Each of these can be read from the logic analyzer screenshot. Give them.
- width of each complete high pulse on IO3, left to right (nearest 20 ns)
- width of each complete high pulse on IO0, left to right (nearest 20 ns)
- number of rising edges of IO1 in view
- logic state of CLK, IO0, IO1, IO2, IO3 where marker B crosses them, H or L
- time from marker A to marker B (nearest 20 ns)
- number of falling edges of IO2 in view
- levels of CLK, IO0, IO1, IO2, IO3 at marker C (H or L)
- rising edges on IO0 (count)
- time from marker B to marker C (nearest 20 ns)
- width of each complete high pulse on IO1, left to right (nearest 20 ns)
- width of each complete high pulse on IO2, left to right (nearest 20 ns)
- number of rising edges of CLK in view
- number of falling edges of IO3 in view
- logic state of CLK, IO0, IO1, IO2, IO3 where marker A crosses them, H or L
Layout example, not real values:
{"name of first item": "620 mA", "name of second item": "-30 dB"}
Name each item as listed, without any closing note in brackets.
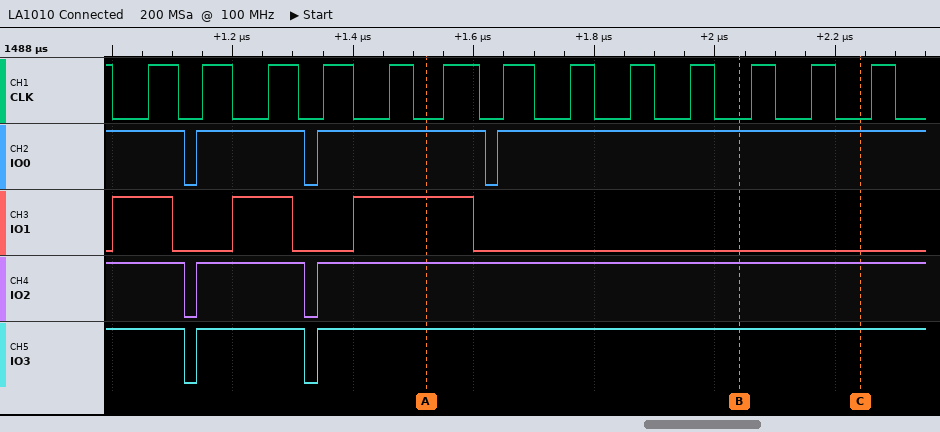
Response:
{"width of each complete high pulse on IO3, left to right": "180 ns", "width of each complete high pulse on IO0, left to right": "180 ns, 280 ns", "number of rising edges of IO1 in view": "3", "logic state of CLK, IO0, IO1, IO2, IO3 where marker B crosses them, H or L": "CLK=L, IO0=H, IO1=L, IO2=H, IO3=H", "time from marker A to marker B": "520 ns", "number of falling edges of IO2 in view": "2", "levels of CLK, IO0, IO1, IO2, IO3 at marker C": "CLK=L, IO0=H, IO1=L, IO2=H, IO3=H", "rising edges on IO0": "3", "time from marker B to marker C": "200 ns", "width of each complete high pulse on IO1, left to right": "100 ns, 100 ns, 200 ns", "width of each complete high pulse on IO2, left to right": "180 ns", "number of rising edges of CLK in view": "13", "number of falling edges of IO3 in view": "2", "logic state of CLK, IO0, IO1, IO2, IO3 where marker A crosses them, H or L": "CLK=L, IO0=H, IO1=H, IO2=H, IO3=H"}
